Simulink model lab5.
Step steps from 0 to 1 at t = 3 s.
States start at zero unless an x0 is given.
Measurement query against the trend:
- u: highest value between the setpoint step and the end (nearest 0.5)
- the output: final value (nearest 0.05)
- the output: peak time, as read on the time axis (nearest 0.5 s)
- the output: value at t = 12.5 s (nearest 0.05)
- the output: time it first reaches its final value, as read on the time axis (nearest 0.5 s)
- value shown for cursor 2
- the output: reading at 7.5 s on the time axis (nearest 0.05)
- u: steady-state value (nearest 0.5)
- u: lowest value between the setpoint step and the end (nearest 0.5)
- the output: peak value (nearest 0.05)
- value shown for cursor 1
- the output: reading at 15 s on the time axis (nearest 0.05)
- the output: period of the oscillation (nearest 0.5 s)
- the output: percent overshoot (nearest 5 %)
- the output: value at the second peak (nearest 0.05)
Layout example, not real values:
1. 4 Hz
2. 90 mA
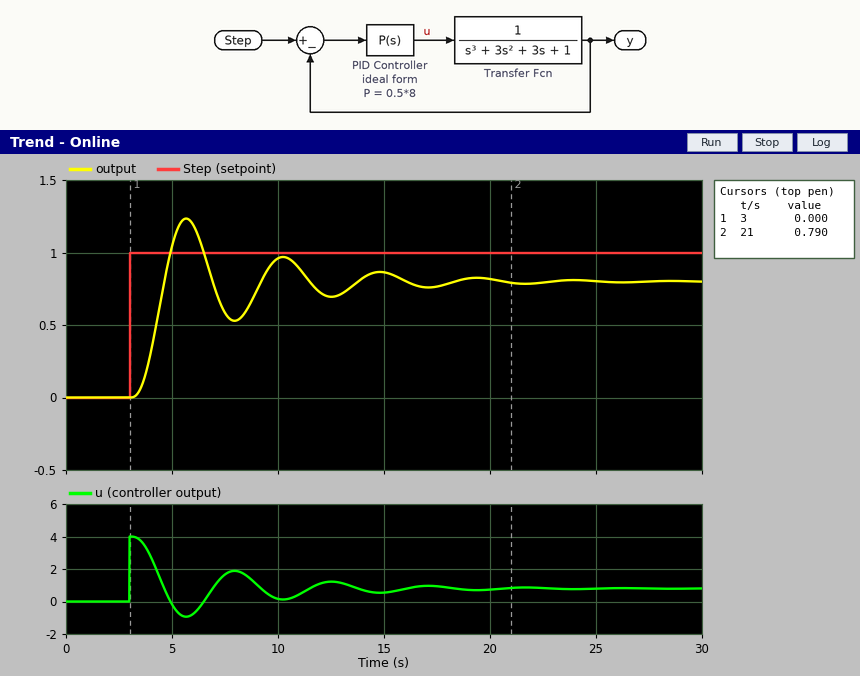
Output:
1. 4.0
2. 0.80
3. 5.5 s
4. 0.70
5. 4.5 s
6. 0.790
7. 0.60
8. 1.0
9. -1.0
10. 1.25
11. 0.000
12. 0.85
13. 4.5 s
14. 55 %
15. 0.95
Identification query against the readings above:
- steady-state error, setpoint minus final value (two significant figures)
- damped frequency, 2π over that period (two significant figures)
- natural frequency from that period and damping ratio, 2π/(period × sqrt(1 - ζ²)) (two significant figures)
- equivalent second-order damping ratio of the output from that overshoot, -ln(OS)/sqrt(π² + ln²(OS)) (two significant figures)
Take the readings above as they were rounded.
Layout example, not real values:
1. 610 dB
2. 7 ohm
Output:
1. 0.20
2. 1.4 rad/s
3. 1.4 rad/s
4. 0.19
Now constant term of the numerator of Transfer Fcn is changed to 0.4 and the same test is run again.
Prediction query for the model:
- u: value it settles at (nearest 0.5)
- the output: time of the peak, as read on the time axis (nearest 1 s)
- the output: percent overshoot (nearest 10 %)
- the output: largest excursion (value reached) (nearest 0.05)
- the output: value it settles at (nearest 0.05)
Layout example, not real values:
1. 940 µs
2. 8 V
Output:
1. 1.5
2. 7 s
3. 20 %
4. 0.75
5. 0.60
